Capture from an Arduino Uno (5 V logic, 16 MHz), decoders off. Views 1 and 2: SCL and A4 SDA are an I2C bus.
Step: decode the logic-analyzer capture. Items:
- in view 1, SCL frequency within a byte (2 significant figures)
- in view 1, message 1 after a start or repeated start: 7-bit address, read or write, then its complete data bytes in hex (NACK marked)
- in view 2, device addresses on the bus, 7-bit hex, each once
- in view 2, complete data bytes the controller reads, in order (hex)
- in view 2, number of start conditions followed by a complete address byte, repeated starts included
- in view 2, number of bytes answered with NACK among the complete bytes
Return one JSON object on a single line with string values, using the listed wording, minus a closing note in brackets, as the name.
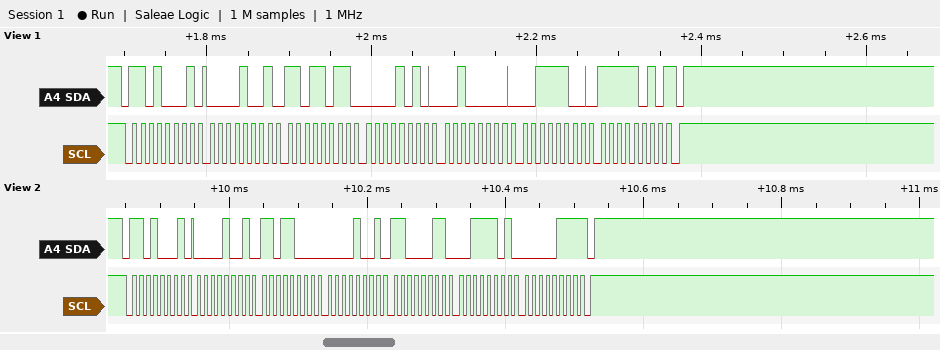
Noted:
{"in view 1, SCL frequency within a byte": "100 kHz", "in view 1, message 1 after a start or repeated start: 7-bit address, read or write, then its complete data bytes in hex": "0x68 read: 09 DB 0A 20 3C FA NACK", "in view 2, device addresses on the bus, 7-bit hex, each once": "0x68", "in view 2, complete data bytes the controller reads, in order": "09 D8 09 C3 3D 07", "in view 2, number of start conditions followed by a complete address byte, repeated starts included": "1", "in view 2, number of bytes answered with NACK among the complete bytes": "1"}
